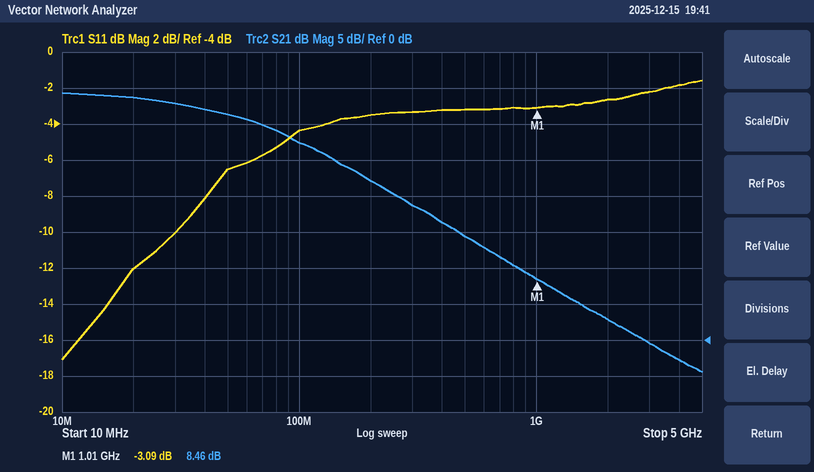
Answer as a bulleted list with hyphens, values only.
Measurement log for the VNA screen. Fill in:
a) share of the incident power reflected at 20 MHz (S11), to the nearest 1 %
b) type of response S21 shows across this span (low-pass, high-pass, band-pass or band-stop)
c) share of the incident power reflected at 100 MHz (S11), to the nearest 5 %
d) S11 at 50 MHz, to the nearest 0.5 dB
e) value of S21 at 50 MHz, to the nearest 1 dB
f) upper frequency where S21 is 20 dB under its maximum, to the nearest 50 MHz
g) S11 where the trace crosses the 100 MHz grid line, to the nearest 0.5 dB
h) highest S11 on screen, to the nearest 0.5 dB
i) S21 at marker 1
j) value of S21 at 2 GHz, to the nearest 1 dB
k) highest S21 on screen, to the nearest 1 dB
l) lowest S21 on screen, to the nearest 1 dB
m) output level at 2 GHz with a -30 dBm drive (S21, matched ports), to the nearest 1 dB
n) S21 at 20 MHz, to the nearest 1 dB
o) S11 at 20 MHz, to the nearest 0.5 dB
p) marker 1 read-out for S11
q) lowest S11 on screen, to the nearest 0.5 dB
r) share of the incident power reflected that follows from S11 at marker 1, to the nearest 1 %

- 6 %
- low-pass
- 35 %
- -6.5 dB
- 31 dB
- 500 MHz
- -4.5 dB
- -1.5 dB
- 8.46 dB
- 3 dB
- 34 dB
- -4 dB
- -27 dBm
- 34 dB
- -12.0 dB
- -3.09 dB
- -17.0 dB
- 49 %
